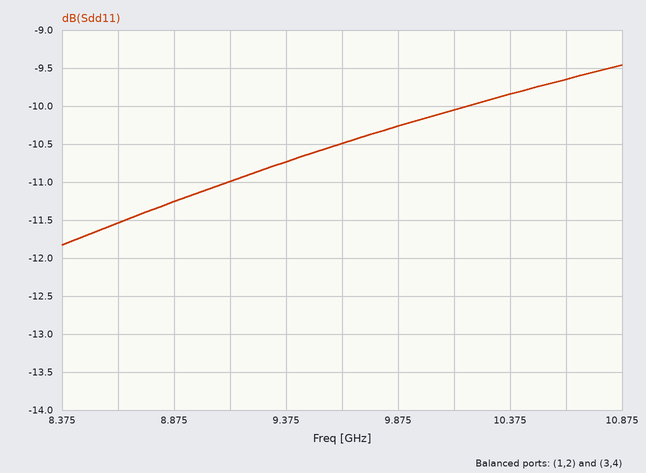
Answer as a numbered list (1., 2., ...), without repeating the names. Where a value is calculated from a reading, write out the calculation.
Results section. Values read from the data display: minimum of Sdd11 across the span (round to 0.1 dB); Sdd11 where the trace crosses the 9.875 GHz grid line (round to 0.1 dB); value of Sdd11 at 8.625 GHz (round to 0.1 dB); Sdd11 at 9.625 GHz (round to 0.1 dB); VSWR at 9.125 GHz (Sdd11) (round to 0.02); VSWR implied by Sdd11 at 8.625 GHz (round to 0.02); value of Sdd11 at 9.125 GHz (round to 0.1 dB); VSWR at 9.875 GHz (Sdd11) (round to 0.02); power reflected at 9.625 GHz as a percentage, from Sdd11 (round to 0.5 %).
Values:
1. -11.8 dB
2. -10.3 dB
3. -11.5 dB
4. -10.5 dB
5. |Γ| = 10^(-11/20) = 0.2818; VSWR = (1 + 0.2818)/(1 − 0.2818) ≈ 1.78
6. |Γ| = 10^(-11.5/20) = 0.2661; VSWR = (1 + 0.2661)/(1 − 0.2661) ≈ 1.73, so 1.72 to the nearest 0.02
7. -11.0 dB
8. |Γ| = 10^(-10.3/20) = 0.3055; VSWR = (1 + 0.3055)/(1 − 0.3055) ≈ 1.88
9. 10^(-10.5/10) ≈ 8.91 %, so 9.0 % to the nearest 0.5 %
